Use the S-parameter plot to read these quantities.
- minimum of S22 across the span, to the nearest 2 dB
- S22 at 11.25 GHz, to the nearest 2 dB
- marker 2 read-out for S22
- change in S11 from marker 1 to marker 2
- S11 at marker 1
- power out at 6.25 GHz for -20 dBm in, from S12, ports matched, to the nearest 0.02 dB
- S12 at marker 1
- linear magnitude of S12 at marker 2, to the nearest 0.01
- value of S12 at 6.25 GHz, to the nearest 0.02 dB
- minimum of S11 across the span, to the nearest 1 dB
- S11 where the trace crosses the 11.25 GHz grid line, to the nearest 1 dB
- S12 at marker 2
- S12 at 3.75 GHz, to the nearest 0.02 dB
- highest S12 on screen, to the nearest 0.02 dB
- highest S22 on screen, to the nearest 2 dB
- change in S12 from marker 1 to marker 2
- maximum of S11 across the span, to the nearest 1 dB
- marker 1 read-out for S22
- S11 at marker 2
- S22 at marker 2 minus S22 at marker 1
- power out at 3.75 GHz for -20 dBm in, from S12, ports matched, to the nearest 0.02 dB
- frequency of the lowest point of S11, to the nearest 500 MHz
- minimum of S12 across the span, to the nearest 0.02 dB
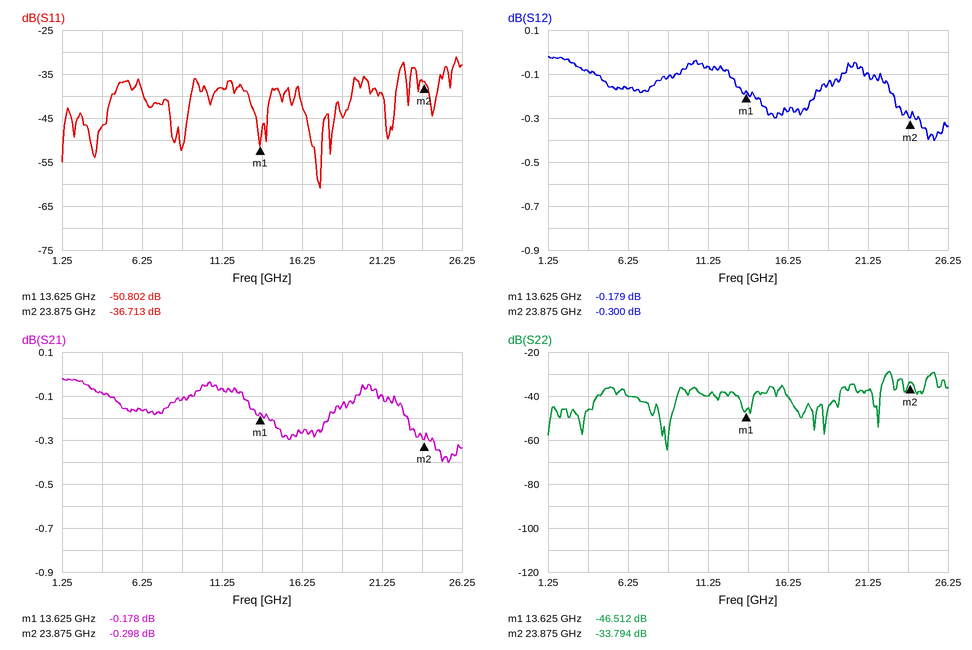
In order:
-64 dB
-40 dB
-33.794 dB
14.089 dB
-50.802 dB
-20.16 dBm
-0.179 dB
0.97
-0.16 dB
-61 dB
-38 dB
-0.300 dB
-0.08 dB
-0.02 dB
-28 dB
-0.121 dB
-31 dB
-46.512 dB
-36.713 dB
12.718 dB
-20.08 dBm
17.5 GHz
-0.40 dB
